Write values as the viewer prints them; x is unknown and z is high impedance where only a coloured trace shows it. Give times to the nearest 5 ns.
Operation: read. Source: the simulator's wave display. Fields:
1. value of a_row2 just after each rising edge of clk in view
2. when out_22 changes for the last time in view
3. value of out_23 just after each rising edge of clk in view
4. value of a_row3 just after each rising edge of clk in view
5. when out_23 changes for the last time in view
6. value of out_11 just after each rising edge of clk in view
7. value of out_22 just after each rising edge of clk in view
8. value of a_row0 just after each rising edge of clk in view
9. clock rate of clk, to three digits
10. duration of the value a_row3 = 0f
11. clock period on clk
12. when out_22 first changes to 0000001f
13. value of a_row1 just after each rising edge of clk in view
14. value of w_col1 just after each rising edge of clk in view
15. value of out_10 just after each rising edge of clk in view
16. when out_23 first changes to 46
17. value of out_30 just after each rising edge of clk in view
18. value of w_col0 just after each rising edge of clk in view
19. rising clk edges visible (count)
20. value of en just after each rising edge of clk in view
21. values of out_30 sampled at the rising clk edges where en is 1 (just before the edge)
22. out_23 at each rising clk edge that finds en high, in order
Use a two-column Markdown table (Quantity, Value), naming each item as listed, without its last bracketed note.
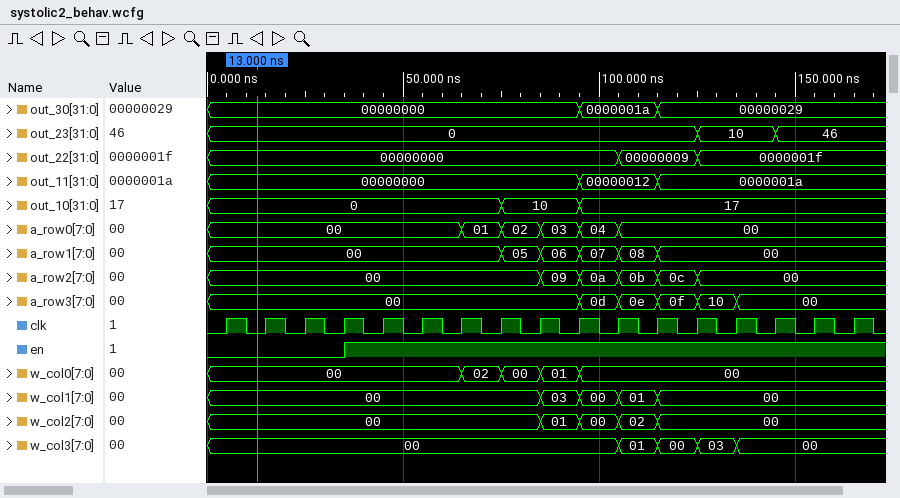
| Quantity | Value |
|---|---|
| value of a_row2 just after each rising edge of clk in view | 00, 00, 00, 00, 00, 00, 00, 00, 09, 0a, 0b, 0c, 00, 00, 00, 00, 00 |
| when out_22 changes for the last time in view | 125 ns |
| value of out_23 just after each rising edge of clk in view | 0, 0, 0, 0, 0, 0, 0, 0, 0, 0, 0, 0, 10, 10, 46, 46, 46 |
| value of a_row3 just after each rising edge of clk in view | 00, 00, 00, 00, 00, 00, 00, 00, 00, 0d, 0e, 0f, 10, 00, 00, 00, 00 |
| when out_23 changes for the last time in view | 145 ns |
| value of out_11 just after each rising edge of clk in view | 00000000, 00000000, 00000000, 00000000, 00000000, 00000000, 00000000, 00000000, 00000000, 00000012, 00000012, 0000001a, 0000001a, 0000001a, 0000001a, 0000001a, 0000001a |
| value of out_22 just after each rising edge of clk in view | 00000000, 00000000, 00000000, 00000000, 00000000, 00000000, 00000000, 00000000, 00000000, 00000000, 00000009, 00000009, 0000001f, 0000001f, 0000001f, 0000001f, 0000001f |
| value of a_row0 just after each rising edge of clk in view | 00, 00, 00, 00, 00, 00, 01, 02, 03, 04, 00, 00, 00, 00, 00, 00, 00 |
| clock rate of clk, to three digits | 100 MHz |
| duration of the value a_row3 = 0f | 10 ns |
| clock period on clk | 10 ns |
| when out_22 first changes to 0000001f | 125 ns |
| value of a_row1 just after each rising edge of clk in view | 00, 00, 00, 00, 00, 00, 00, 05, 06, 07, 08, 00, 00, 00, 00, 00, 00 |
| value of w_col1 just after each rising edge of clk in view | 00, 00, 00, 00, 00, 00, 00, 00, 03, 00, 01, 00, 00, 00, 00, 00, 00 |
| value of out_10 just after each rising edge of clk in view | 0, 0, 0, 0, 0, 0, 0, 10, 10, 17, 17, 17, 17, 17, 17, 17, 17 |
| when out_23 first changes to 46 | 145 ns |
| value of out_30 just after each rising edge of clk in view | 00000000, 00000000, 00000000, 00000000, 00000000, 00000000, 00000000, 00000000, 00000000, 0000001a, 0000001a, 00000029, 00000029, 00000029, 00000029, 00000029, 00000029 |
| value of w_col0 just after each rising edge of clk in view | 00, 00, 00, 00, 00, 00, 02, 00, 01, 00, 00, 00, 00, 00, 00, 00, 00 |
| rising clk edges visible | 17 |
| value of en just after each rising edge of clk in view | 0 0 0 1 1 1 1 1 1 1 1 1 1 1 1 1 1 |
| values of out_30 sampled at the rising clk edges where en is 1 | 00000000, 00000000, 00000000, 00000000, 00000000, 00000000, 0000001a, 0000001a, 00000029, 00000029, 00000029, 00000029, 00000029 |
| out_23 at each rising clk edge that finds en high, in order | 0, 0, 0, 0, 0, 0, 0, 0, 0, 10, 10, 46, 46 |
